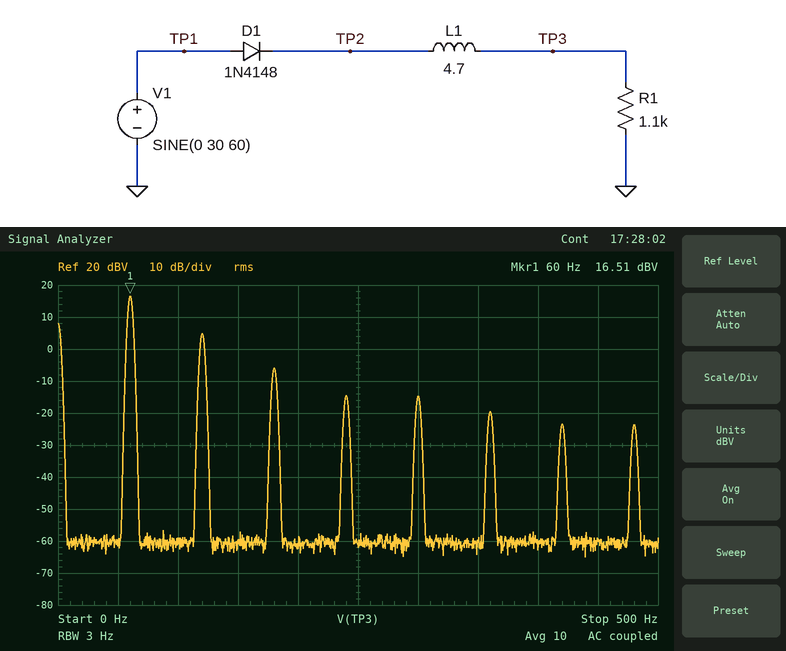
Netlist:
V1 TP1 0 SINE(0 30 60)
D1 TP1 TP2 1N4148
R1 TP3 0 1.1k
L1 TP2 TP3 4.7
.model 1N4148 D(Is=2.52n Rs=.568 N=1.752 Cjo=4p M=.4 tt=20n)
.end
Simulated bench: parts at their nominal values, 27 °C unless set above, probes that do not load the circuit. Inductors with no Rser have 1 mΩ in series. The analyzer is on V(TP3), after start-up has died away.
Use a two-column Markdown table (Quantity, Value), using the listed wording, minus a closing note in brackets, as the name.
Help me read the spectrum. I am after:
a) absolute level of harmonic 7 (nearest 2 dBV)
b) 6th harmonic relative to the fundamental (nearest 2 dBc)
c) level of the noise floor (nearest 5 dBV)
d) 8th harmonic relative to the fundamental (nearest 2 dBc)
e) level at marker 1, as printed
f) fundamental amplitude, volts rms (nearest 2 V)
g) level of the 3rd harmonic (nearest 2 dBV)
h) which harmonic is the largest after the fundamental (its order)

| Quantity | Value |
|---|---|
| absolute level of harmonic 7 | -24 dBV |
| 6th harmonic relative to the fundamental | -36 dBc |
| level of the noise floor | -60 dBV |
| 8th harmonic relative to the fundamental | -40 dBc |
| level at marker 1, as printed | 16.51 dBV |
| fundamental amplitude, volts rms | 6 V |
| level of the 3rd harmonic | -6 dBV |
| which harmonic is the largest after the fundamental | 2 |
